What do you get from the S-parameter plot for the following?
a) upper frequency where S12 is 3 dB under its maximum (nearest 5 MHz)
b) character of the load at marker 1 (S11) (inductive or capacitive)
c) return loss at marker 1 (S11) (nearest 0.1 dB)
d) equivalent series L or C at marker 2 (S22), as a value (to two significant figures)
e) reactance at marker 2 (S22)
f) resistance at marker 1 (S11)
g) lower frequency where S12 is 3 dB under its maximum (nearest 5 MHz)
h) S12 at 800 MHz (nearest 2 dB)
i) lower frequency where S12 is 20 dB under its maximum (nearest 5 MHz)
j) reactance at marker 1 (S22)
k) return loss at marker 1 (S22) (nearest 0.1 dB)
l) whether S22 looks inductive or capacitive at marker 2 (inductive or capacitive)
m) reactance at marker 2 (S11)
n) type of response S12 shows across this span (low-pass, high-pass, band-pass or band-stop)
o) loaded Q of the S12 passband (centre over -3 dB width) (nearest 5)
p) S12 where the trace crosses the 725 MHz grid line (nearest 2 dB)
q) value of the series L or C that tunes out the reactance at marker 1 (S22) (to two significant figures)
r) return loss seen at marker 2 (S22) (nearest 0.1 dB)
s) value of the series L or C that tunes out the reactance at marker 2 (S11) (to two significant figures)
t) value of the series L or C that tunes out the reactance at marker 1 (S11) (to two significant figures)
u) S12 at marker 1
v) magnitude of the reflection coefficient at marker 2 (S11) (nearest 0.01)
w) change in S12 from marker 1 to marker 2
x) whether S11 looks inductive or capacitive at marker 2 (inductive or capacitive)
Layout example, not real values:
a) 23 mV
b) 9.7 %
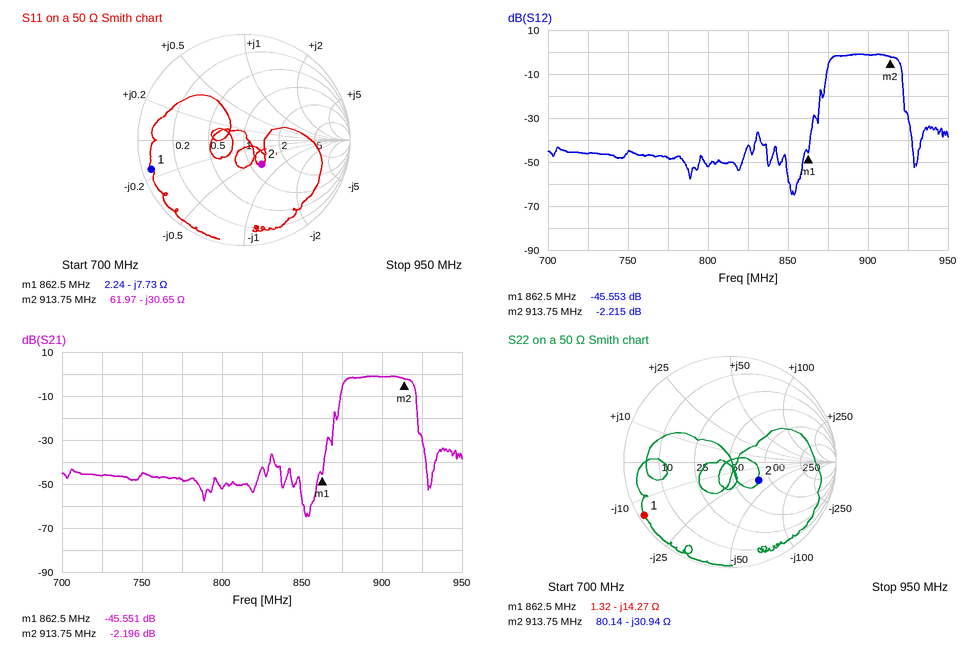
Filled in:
a) 920 MHz
b) capacitive
c) 0.8 dB
d) 5.6 pF
e) -30.94 Ω
f) 2.24 Ω
g) 875 MHz
h) -52 dB
i) 870 MHz
j) -14.27 Ω
k) 0.4 dB
l) capacitive
m) -30.65 Ω
n) band-pass
o) 20
p) -46 dB
q) 2.6 nH
r) 9.8 dB
s) 5.3 nH
t) 1.4 nH
u) -45.553 dB
v) 0.28
w) 43.338 dB
x) capacitive
